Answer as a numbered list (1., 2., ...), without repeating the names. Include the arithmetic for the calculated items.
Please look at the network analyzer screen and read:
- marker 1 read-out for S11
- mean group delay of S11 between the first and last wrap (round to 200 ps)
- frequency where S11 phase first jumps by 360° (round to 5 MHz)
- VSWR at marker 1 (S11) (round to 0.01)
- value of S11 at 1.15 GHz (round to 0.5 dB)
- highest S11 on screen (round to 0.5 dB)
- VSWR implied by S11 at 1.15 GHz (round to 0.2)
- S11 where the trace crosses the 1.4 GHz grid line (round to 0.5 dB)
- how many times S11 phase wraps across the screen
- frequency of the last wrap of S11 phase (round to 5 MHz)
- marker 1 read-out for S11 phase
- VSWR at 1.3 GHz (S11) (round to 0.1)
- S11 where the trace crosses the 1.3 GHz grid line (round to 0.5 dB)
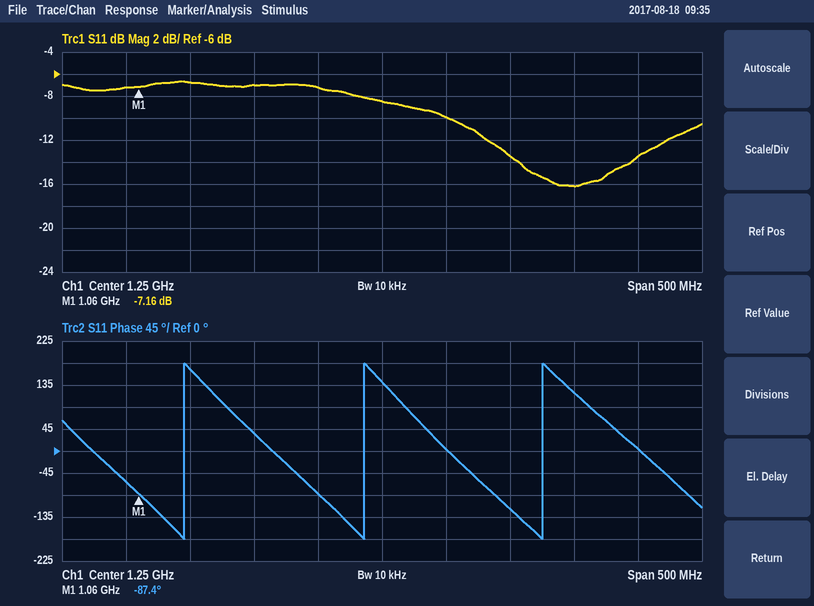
1. -7.16 dB
2. 2 cycles / (1.375 GHz − 1.095 GHz) ≈ 7.14 ns, so 7.2 ns to the nearest 200 ps
3. 1.095 GHz
4. (1 + 0.4385)/(1 − 0.4385) ≈ 2.56
5. -7.0 dB
6. -6.5 dB
7. |Γ| = 10^(-7/20) = 0.4467; VSWR = (1 + 0.4467)/(1 − 0.4467) ≈ 2.6
8. -16.0 dB
9. 3
10. 1.375 GHz
11. -87.4°
12. |Γ| = 10^(-10/20) = 0.3162; VSWR = (1 + 0.3162)/(1 − 0.3162) ≈ 1.9
13. -10.0 dB
